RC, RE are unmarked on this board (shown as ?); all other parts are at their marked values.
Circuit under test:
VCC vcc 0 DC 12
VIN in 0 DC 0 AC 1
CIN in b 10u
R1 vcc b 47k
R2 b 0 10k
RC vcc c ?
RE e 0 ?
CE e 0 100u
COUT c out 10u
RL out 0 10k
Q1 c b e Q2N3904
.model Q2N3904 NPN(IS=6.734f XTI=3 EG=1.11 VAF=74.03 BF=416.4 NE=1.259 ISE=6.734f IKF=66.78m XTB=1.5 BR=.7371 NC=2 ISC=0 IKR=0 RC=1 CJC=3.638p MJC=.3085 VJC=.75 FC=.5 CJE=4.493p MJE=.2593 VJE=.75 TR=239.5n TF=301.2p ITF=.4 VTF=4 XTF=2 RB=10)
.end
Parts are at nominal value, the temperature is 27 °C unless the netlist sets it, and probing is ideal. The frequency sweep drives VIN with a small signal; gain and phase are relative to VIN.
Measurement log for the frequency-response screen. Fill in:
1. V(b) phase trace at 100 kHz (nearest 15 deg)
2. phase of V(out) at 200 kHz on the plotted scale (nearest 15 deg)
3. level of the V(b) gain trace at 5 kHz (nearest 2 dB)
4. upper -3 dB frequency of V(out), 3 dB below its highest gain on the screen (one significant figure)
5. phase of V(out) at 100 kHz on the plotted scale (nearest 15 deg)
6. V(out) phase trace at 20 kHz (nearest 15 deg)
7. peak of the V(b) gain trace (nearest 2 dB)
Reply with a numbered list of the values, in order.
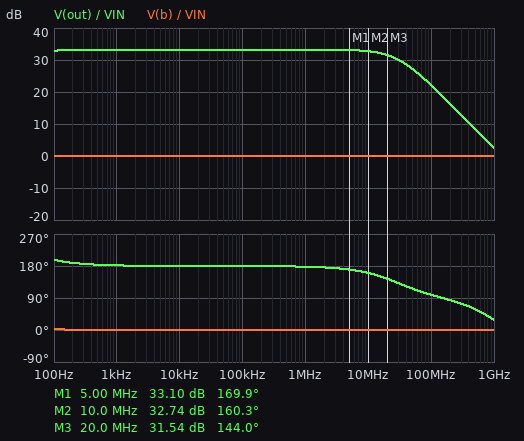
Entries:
1. 0 deg
2. 180 deg
3. 0 dB
4. 30 MHz
5. 180 deg
6. 180 deg
7. 0 dB
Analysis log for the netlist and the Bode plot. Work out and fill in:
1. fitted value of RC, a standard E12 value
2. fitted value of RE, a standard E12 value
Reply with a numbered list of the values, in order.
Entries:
1. 3.9 kΩ
2. 3.3 kΩ
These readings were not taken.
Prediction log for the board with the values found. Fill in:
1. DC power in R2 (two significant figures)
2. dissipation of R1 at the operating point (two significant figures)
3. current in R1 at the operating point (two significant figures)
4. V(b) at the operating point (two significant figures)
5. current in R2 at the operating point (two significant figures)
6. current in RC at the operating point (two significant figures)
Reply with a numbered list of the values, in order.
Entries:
1. 430 µW
2. 2.1 mW
3. 210 µA
4. 2.1 V
5. 210 µA
6. 430 µA
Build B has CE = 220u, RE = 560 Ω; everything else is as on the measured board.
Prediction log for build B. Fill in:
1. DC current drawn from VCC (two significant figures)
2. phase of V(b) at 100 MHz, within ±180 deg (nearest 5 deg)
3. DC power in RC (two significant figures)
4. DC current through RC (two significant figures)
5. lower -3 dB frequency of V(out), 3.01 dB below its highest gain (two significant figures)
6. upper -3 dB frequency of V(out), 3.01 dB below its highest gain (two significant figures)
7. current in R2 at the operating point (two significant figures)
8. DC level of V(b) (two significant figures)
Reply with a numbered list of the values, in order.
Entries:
1. 2.5 mA
2. 0 deg
3. 20 mW
4. 2.3 mA
5. 67 Hz
6. 12 MHz
7. 200 µA
8. 2.0 V
